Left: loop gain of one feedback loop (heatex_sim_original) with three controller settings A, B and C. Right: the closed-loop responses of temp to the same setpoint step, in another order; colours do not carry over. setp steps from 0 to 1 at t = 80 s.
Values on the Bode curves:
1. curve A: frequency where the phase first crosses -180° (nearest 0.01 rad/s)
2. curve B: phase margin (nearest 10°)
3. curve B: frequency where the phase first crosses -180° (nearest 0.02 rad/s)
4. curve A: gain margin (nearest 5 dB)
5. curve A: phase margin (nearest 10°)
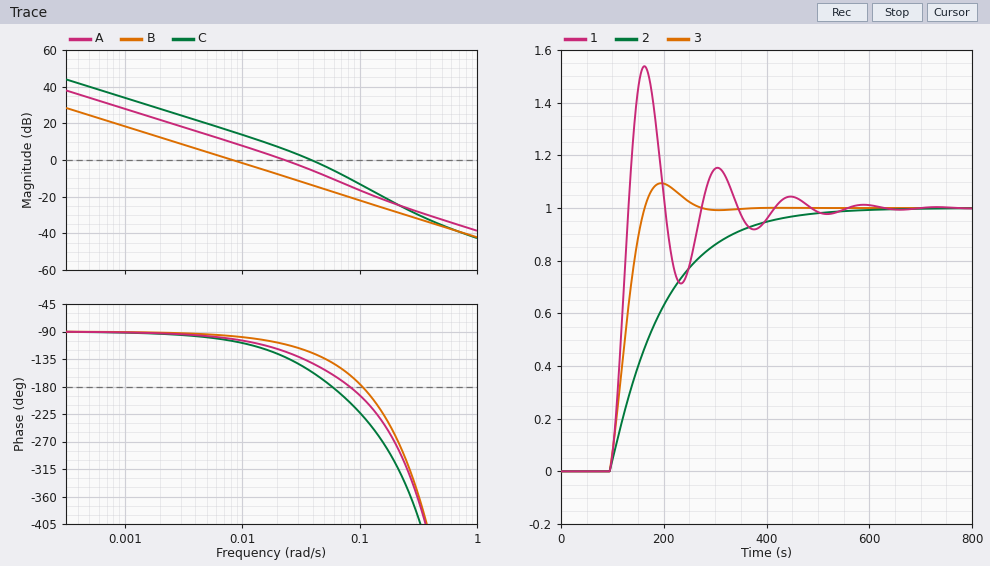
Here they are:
0.08 rad/s
80°
0.10 rad/s
15 dB
60°
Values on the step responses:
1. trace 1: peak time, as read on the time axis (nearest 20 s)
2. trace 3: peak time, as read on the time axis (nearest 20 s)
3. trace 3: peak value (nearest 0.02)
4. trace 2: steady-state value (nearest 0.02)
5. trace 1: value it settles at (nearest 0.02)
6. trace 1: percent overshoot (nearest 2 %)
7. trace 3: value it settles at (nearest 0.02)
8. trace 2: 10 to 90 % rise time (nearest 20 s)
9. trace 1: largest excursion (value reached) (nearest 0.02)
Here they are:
160 s
200 s
1.10
1.00
1.00
54 %
1.00
220 s
1.54
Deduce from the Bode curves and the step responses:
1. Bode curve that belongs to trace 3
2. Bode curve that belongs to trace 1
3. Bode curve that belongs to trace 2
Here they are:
A
C
B
